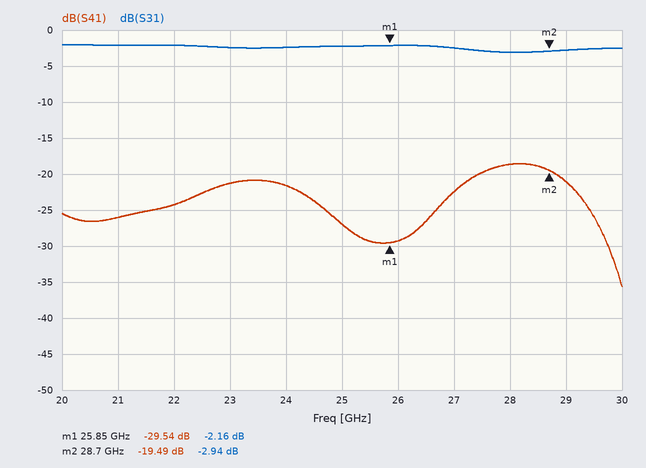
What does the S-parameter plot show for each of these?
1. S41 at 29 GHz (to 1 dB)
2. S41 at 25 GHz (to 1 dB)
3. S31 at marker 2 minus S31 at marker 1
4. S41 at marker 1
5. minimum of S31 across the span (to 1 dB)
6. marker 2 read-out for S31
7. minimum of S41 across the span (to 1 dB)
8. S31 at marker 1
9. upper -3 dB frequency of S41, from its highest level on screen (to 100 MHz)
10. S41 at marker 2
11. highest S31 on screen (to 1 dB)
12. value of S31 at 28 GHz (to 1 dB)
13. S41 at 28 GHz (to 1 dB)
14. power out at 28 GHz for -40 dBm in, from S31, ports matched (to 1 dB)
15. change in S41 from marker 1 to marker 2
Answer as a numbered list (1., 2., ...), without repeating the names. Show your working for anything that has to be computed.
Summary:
1. -21 dB
2. -27 dB
3. -2.94 − (-2.16) = -0.78 dB
4. -29.54 dB
5. -3 dB
6. -2.94 dB
7. -36 dB
8. -2.16 dB
9. 29.1 GHz
10. -19.49 dB
11. -2 dB
12. -3 dB
13. -19 dB
14. -40 dBm + (-3 dB) = -43 dBm
15. -19.49 − (-29.54) = 10.05 dB
